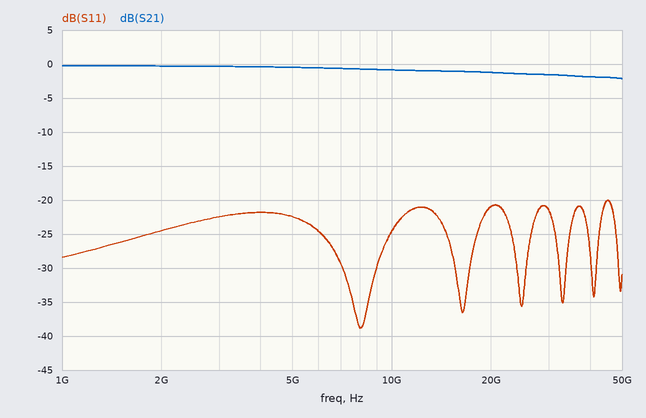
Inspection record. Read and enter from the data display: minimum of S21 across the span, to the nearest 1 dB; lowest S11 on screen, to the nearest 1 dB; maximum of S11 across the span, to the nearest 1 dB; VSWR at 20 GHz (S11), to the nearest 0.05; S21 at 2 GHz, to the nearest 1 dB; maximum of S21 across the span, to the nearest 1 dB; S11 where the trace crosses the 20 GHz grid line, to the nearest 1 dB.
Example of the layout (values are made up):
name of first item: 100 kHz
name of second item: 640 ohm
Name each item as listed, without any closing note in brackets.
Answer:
minimum of S21 across the span, to the nearest 1 dB: -2 dB
lowest S11 on screen, to the nearest 1 dB: -39 dB
maximum of S11 across the span, to the nearest 1 dB: -20 dB
VSWR at 20 GHz (S11), to the nearest 0.05: 1.20
S21 at 2 GHz, to the nearest 1 dB: 0 dB
maximum of S21 across the span, to the nearest 1 dB: 0 dB
S11 where the trace crosses the 20 GHz grid line, to the nearest 1 dB: -21 dB
